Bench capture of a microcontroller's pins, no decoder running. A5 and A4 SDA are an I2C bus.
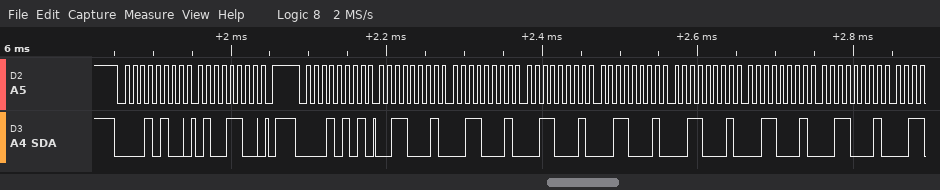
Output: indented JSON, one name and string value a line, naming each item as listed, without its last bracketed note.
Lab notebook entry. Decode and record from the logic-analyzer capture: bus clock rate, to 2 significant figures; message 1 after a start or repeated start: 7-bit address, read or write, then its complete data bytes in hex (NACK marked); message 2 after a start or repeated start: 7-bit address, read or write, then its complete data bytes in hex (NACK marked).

{
  "bus clock rate, to 2 significant figures": "100 kHz",
  "message 1 after a start or repeated start: 7-bit address, read or write, then its complete data bytes in hex": "0x0A write: 4C",
  "message 2 after a start or repeated start: 7-bit address, read or write, then its complete data bytes in hex": "0x0A read: 31 31 31 31 31 31 31"
}
